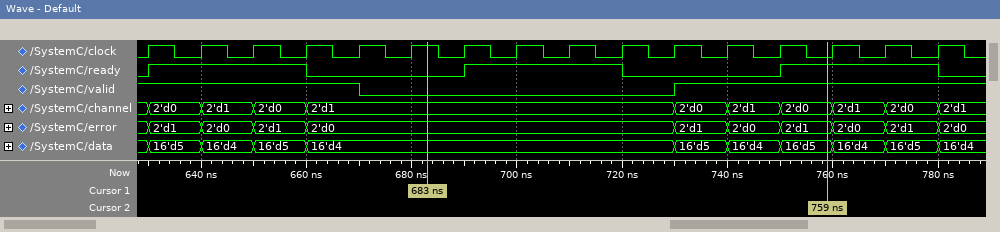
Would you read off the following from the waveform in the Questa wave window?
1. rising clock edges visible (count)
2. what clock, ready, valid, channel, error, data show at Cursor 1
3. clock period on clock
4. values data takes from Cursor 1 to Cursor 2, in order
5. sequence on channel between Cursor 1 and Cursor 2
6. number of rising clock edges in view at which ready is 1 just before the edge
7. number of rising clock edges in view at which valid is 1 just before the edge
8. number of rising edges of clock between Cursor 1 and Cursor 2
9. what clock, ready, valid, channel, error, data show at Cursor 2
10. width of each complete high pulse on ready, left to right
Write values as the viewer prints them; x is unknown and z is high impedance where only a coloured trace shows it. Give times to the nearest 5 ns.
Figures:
16
clock=1, ready=0, valid=0, channel=2'd1, error=2'd0, data=16'd4
10 ns
16'd4, 16'd5, 16'd4, 16'd5
2'd1, 2'd0, 2'd1, 2'd0
9
10
7
clock=0, ready=1, valid=1, channel=2'd0, error=2'd1, data=16'd5
30 ns, 30 ns, 30 ns
